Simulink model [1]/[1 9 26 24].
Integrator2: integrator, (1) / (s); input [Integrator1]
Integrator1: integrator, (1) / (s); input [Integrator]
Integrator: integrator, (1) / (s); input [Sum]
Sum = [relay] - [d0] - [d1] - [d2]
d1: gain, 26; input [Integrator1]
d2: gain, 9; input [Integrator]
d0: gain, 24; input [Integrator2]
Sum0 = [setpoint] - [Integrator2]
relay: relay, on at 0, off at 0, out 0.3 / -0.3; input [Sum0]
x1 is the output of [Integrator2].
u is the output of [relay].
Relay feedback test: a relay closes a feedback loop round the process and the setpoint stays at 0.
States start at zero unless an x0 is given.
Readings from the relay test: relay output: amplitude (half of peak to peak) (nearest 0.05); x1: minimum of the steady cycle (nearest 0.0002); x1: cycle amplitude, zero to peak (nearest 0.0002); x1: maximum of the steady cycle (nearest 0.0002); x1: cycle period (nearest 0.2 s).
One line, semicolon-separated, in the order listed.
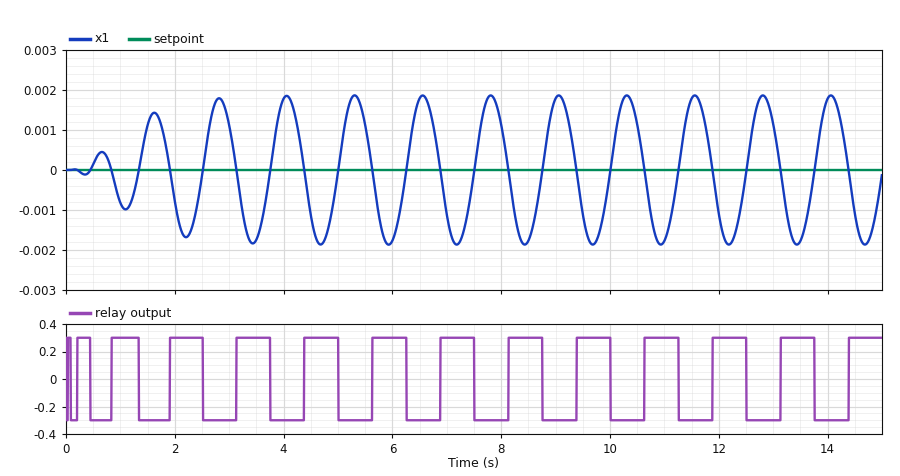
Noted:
0.30; -0.0018; 0.0018; 0.0018; 1.2 s
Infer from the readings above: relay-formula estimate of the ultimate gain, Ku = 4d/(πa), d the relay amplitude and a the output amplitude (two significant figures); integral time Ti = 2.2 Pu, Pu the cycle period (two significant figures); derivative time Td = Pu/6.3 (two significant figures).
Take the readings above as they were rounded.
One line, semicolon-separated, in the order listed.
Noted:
210; 2.6 s; 0.19 s
